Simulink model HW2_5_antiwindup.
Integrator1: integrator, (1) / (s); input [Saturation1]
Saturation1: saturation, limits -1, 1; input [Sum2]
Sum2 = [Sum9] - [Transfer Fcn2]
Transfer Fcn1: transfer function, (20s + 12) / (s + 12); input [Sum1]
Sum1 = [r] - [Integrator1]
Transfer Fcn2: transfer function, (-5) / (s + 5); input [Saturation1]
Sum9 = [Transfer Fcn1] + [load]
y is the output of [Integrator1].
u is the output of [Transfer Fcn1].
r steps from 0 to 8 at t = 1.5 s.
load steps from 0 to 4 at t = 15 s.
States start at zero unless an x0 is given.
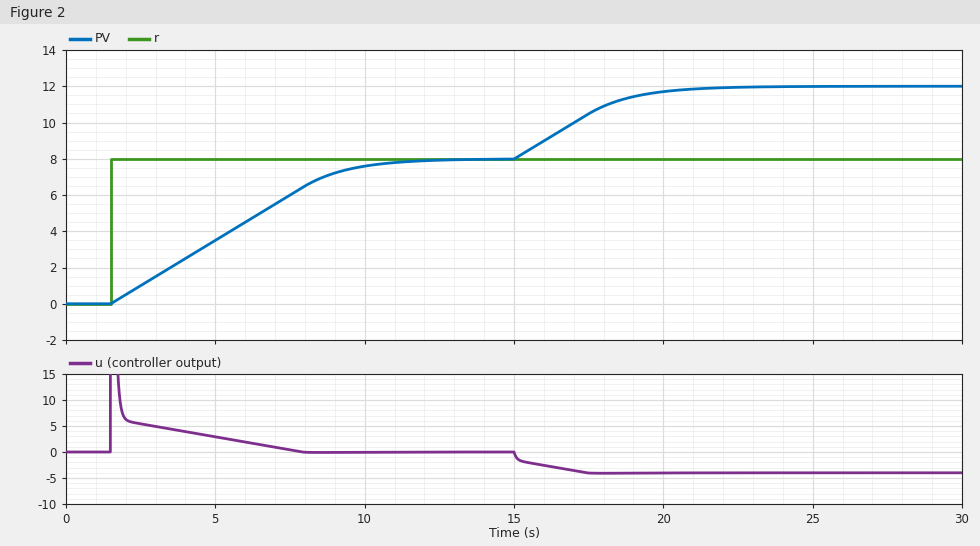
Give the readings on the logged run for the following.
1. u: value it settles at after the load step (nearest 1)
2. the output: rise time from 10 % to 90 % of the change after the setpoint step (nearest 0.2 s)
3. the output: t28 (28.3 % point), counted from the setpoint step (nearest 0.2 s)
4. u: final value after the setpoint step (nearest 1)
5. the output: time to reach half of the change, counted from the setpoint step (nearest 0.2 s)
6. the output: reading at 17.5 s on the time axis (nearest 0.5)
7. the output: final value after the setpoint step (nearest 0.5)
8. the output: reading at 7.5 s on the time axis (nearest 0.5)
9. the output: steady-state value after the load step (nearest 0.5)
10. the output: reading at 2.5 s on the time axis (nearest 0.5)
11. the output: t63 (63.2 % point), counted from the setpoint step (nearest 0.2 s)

-4
6.6 s
2.2 s
0
4.0 s
10.5
8.0
6.0
12.0
1.0
5.0 s
